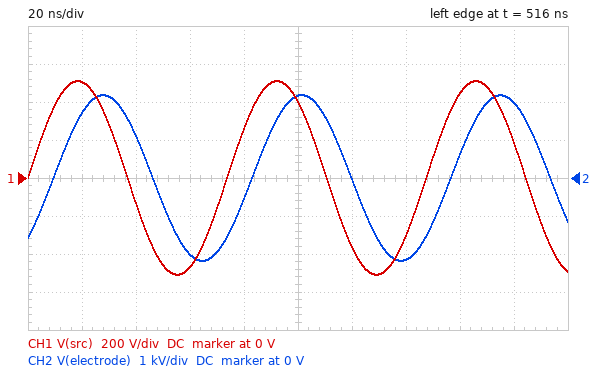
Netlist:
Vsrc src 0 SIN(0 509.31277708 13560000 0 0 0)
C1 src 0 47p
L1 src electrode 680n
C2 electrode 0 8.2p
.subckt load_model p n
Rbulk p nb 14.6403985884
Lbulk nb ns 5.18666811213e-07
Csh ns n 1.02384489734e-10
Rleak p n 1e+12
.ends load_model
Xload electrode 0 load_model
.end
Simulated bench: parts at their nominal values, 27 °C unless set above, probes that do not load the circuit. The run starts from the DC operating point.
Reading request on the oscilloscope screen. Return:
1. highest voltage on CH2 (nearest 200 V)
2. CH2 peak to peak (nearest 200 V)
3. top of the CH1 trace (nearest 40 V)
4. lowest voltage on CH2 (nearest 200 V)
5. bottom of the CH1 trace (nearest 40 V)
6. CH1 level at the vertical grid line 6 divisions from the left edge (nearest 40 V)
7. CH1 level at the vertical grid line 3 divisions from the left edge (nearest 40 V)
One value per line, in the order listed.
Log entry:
2.2 kV
4.4 kV
520 V
-2.2 kV
-520 V
-360 V
-480 V
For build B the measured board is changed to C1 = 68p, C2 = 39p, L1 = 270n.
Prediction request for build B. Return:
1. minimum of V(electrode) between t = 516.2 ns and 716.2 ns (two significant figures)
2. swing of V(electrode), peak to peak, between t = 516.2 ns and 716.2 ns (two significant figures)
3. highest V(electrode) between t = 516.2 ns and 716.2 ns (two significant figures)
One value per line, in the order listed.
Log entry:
-830 V
1.7 kV
830 V
